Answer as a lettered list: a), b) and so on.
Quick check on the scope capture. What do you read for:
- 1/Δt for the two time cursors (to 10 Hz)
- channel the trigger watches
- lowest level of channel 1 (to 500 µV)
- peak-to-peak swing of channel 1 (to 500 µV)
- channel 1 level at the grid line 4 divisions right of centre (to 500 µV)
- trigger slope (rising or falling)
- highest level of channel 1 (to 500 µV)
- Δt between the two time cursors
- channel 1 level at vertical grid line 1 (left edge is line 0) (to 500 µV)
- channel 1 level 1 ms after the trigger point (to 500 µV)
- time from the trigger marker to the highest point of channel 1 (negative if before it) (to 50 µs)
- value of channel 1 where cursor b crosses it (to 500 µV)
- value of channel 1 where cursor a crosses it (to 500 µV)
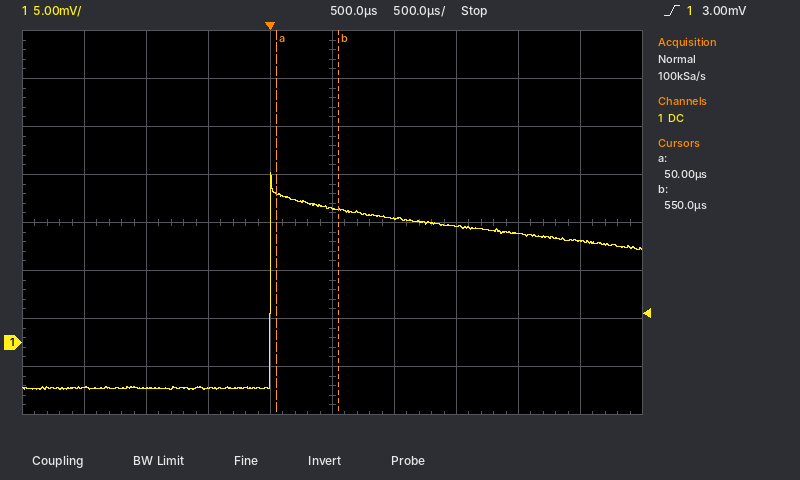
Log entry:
a) 2.00 kHz
b) channel 1
c) -5.0 mV
d) 22.5 mV
e) 10.5 mV
f) rising
g) 17.5 mV
h) 500 µs
i) -4.5 mV
j) 13.0 mV
k) 0 µs
l) 14.0 mV
m) 15.5 mV
